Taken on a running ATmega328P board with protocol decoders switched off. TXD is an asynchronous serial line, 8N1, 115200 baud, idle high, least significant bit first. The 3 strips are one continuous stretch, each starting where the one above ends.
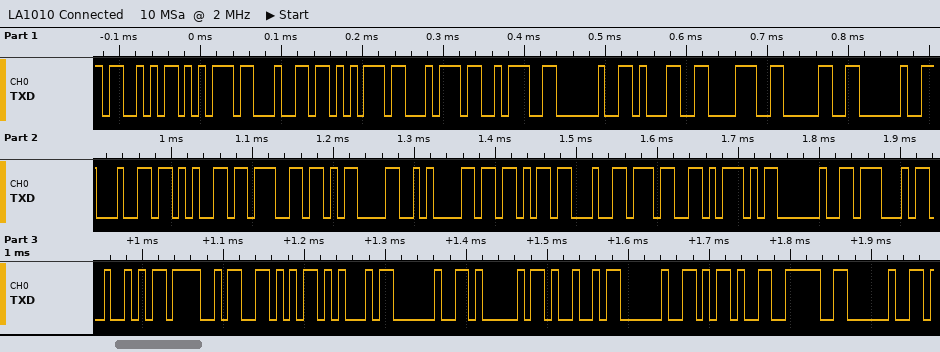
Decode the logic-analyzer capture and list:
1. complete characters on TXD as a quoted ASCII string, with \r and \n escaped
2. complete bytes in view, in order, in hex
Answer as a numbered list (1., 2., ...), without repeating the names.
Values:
1. "Sudut: 180 deg\r\n[#7] GROVE AI -> "
2. 53 75 64 75 74 3A 20 31 38 30 20 64 65 67 0D 0A 5B 23 37 5D 20 47 52 4F 56 45 20 41 49 20 2D 3E 20
